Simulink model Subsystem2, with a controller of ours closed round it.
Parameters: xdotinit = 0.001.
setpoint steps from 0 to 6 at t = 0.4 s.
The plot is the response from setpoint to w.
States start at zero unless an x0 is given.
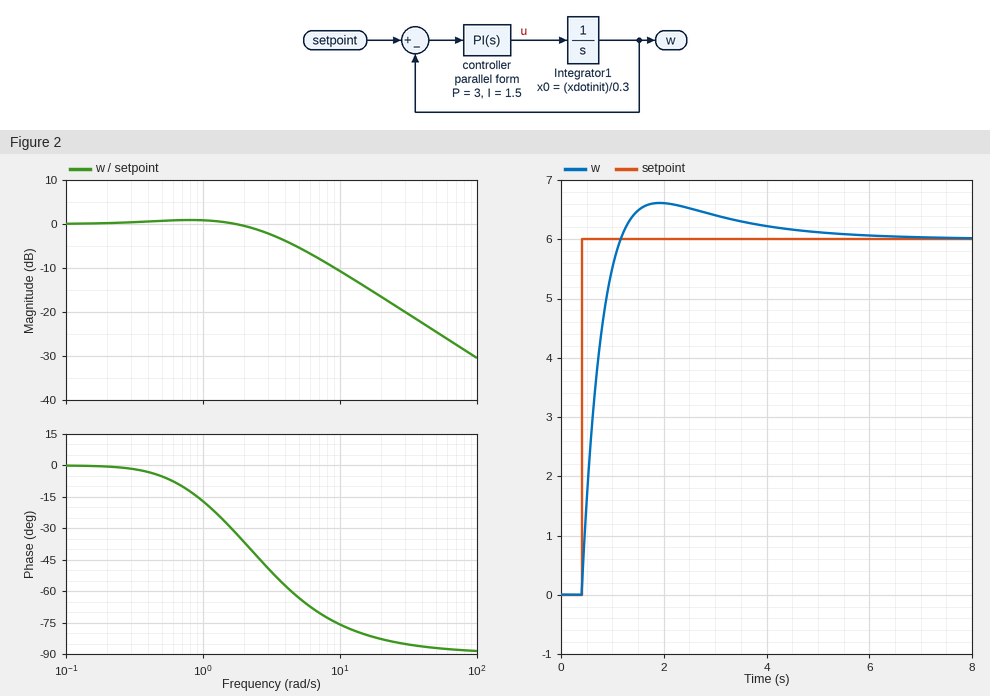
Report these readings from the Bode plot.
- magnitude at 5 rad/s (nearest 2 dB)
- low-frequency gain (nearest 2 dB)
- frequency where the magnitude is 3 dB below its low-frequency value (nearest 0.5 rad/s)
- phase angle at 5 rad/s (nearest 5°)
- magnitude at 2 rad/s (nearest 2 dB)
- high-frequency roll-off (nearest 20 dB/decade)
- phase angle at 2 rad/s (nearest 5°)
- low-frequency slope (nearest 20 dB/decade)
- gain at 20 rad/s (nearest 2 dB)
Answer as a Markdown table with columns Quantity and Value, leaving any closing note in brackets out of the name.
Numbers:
| Quantity | Value |
|---|---|
| magnitude at 5 rad/s | -6 dB |
| low-frequency gain | 0 dB |
| frequency where the magnitude is 3 dB below its low-frequency value | 3.5 rad/s |
| phase angle at 5 rad/s | -65° |
| magnitude at 2 rad/s | 0 dB |
| high-frequency roll-off | -20 dB/decade |
| phase angle at 2 rad/s | -35° |
| low-frequency slope | 0 dB/decade |
| gain at 20 rad/s | -16 dB |
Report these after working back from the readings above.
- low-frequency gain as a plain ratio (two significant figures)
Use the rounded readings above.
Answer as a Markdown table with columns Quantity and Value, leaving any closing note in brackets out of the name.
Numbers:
| Quantity | Value |
|---|---|
| low-frequency gain as a plain ratio | 1.0 |
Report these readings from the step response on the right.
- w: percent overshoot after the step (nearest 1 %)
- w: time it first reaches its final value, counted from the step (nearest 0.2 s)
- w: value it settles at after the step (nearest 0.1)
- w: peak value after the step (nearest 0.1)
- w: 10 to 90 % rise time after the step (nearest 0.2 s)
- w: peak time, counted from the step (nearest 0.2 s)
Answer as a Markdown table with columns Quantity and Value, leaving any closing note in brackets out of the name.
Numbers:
| Quantity | Value |
|---|---|
| w: percent overshoot after the step | 10 % |
| w: time it first reaches its final value, counted from the step | 0.8 s |
| w: value it settles at after the step | 6.0 |
| w: peak value after the step | 6.6 |
| w: 10 to 90 % rise time after the step | 0.6 s |
| w: peak time, counted from the step | 1.6 s |
